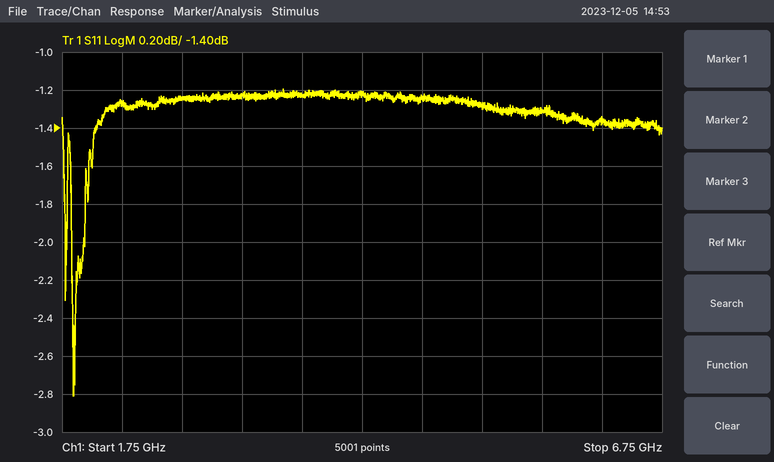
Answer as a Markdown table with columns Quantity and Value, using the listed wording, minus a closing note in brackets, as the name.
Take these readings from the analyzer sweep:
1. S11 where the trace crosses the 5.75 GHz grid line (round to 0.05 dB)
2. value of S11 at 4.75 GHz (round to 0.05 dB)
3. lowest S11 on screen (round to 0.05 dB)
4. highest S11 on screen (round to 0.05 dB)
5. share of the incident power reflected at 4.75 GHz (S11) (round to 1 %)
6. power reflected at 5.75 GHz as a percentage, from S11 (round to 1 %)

| Quantity | Value |
|---|---|
| S11 where the trace crosses the 5.75 GHz grid line | -1.30 dB |
| value of S11 at 4.75 GHz | -1.25 dB |
| lowest S11 on screen | -2.80 dB |
| highest S11 on screen | -1.20 dB |
| share of the incident power reflected at 4.75 GHz (S11) | 75 % |
| power reflected at 5.75 GHz as a percentage, from S11 | 74 % |
